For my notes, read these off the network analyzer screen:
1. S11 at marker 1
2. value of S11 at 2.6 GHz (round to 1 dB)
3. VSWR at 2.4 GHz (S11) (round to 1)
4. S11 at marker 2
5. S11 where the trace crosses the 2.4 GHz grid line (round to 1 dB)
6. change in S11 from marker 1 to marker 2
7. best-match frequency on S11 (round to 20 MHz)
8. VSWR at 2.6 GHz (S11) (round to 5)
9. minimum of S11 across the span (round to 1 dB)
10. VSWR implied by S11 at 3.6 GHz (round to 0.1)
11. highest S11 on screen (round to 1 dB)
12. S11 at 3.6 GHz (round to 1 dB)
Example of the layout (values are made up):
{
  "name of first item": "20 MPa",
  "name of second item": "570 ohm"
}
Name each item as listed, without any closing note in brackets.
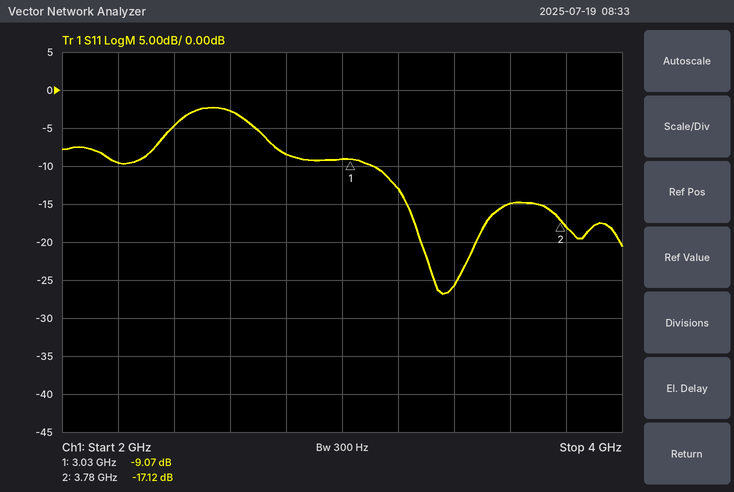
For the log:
{
  "S11 at marker 1": "-9.07 dB",
  "value of S11 at 2.6 GHz": "-3 dB",
  "VSWR at 2.4 GHz (S11)": "4",
  "S11 at marker 2": "-17.12 dB",
  "S11 where the trace crosses the 2.4 GHz grid line": "-5 dB",
  "change in S11 from marker 1 to marker 2": "-8.05 dB",
  "best-match frequency on S11": "3.36 GHz",
  "VSWR at 2.6 GHz (S11)": "5",
  "minimum of S11 across the span": "-27 dB",
  "VSWR implied by S11 at 3.6 GHz": "1.4",
  "highest S11 on screen": "-2 dB",
  "S11 at 3.6 GHz": "-15 dB"
}
